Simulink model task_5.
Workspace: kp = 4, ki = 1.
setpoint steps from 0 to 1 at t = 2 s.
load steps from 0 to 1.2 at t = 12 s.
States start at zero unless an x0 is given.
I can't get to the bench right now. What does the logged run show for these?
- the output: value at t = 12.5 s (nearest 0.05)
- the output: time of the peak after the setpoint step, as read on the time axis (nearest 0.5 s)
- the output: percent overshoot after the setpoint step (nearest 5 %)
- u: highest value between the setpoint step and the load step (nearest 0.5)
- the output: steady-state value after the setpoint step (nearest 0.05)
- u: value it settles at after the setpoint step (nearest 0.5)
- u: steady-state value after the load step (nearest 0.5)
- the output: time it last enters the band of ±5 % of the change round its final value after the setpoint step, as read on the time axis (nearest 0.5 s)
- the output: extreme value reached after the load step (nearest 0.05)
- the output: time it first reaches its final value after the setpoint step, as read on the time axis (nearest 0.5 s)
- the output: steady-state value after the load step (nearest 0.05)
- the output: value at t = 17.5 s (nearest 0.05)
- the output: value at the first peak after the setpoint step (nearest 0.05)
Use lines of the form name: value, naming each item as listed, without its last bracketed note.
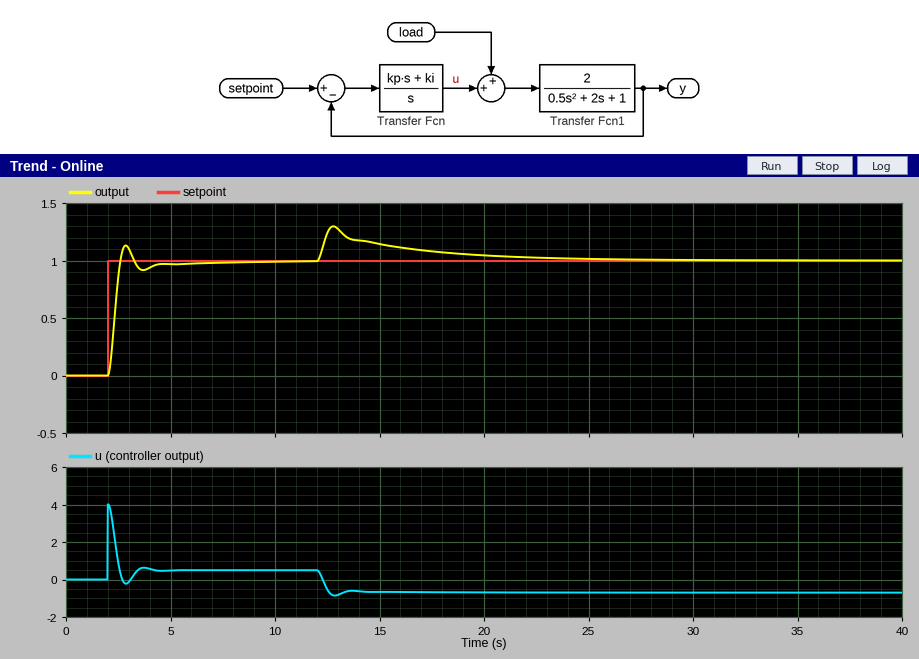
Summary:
the output: value at t = 12.5 s: 1.25
the output: time of the peak after the setpoint step, as read on the time axis: 3.0 s
the output: percent overshoot after the setpoint step: 15 %
u: highest value between the setpoint step and the load step: 4.0
the output: steady-state value after the setpoint step: 1.00
u: value it settles at after the setpoint step: 0.5
u: steady-state value after the load step: -0.5
the output: time it last enters the band of ±5 % of the change round its final value after the setpoint step, as read on the time axis: 4.0 s
the output: extreme value reached after the load step: 1.30
the output: time it first reaches its final value after the setpoint step, as read on the time axis: 2.5 s
the output: steady-state value after the load step: 1.00
the output: value at t = 17.5 s: 1.10
the output: value at the first peak after the setpoint step: 1.15
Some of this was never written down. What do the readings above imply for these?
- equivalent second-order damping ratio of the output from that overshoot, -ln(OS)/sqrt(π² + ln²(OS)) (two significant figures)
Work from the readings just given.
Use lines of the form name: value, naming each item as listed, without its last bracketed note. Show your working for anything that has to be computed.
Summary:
equivalent second-order damping ratio of the output from that overshoot, -ln(OS)/sqrt(π² + ln²(OS)): ln(0.15) = -1.897; 1.897 / sqrt(9.870 + 3.599) = 0.52
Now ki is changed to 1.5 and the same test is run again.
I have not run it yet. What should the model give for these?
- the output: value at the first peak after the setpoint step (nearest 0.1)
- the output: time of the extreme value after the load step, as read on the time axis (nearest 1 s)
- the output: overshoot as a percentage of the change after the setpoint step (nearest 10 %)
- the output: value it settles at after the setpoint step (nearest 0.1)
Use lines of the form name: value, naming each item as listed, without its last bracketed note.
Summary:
the output: value at the first peak after the setpoint step: 1.2
the output: time of the extreme value after the load step, as read on the time axis: 13 s
the output: overshoot as a percentage of the change after the setpoint step: 20 %
the output: value it settles at after the setpoint step: 1.0
